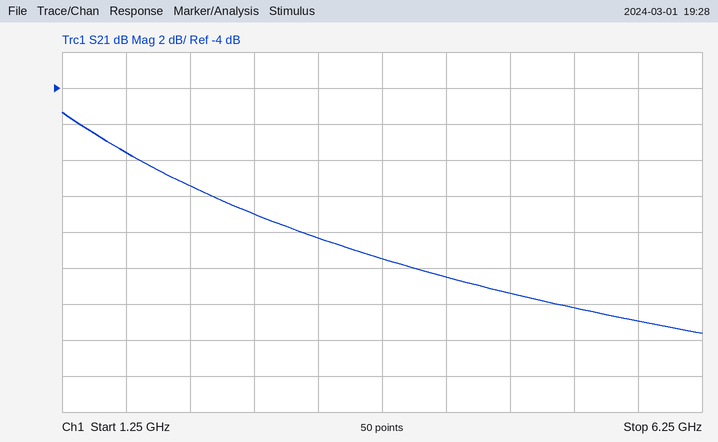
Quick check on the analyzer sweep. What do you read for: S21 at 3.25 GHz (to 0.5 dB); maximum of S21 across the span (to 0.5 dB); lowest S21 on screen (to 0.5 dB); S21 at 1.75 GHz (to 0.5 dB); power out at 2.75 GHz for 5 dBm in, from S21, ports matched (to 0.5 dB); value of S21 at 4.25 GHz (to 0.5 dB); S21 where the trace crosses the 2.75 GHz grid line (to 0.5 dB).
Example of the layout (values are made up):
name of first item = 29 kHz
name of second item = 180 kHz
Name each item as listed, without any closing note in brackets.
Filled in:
S21 at 3.25 GHz = -12.5 dB
maximum of S21 across the span = -5.5 dB
lowest S21 on screen = -17.5 dB
S21 at 1.75 GHz = -7.5 dB
power out at 2.75 GHz for 5 dBm in, from S21, ports matched = -6.0 dBm
value of S21 at 4.25 GHz = -14.5 dB
S21 where the trace crosses the 2.75 GHz grid line = -11.0 dB
